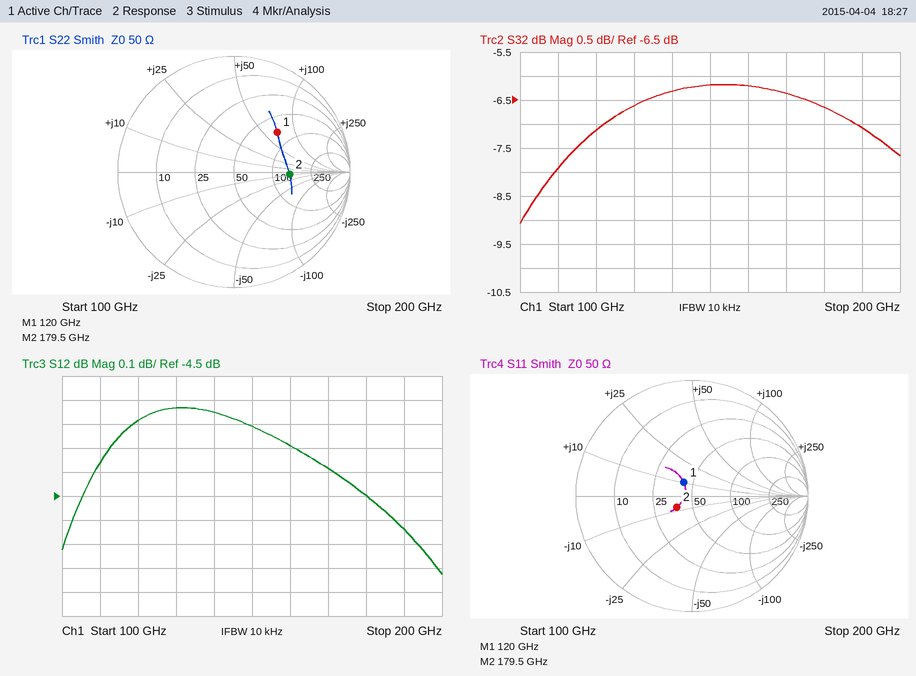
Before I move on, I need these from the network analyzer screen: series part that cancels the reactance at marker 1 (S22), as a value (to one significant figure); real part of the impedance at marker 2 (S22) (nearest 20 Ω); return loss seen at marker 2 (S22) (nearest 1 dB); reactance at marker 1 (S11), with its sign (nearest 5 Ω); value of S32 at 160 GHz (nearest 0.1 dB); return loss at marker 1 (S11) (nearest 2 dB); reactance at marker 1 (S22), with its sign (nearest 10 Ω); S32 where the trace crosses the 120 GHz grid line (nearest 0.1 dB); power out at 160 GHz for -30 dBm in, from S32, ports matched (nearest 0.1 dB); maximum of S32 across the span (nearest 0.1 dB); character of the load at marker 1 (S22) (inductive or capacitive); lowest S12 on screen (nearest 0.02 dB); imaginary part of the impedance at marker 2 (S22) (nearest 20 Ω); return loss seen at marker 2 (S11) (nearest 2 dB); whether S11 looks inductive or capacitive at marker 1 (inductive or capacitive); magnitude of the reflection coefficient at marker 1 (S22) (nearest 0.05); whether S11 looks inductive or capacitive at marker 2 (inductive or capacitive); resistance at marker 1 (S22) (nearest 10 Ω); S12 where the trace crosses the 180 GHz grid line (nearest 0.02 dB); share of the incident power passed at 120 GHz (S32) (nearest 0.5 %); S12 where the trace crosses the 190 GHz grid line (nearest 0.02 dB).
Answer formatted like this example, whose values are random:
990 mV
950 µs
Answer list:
20 fF
140 Ω
6 dB
+10 Ω
-6.2 dB
18 dB
+70 Ω
-7.1 dB
-36.2 dBm
-6.2 dB
inductive
-4.82 dB
0 Ω
16 dB
inductive
0.50
capacitive
70 Ω
-4.50 dB
19.5 %
-4.64 dB
